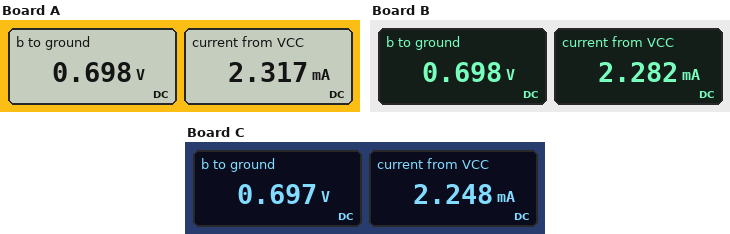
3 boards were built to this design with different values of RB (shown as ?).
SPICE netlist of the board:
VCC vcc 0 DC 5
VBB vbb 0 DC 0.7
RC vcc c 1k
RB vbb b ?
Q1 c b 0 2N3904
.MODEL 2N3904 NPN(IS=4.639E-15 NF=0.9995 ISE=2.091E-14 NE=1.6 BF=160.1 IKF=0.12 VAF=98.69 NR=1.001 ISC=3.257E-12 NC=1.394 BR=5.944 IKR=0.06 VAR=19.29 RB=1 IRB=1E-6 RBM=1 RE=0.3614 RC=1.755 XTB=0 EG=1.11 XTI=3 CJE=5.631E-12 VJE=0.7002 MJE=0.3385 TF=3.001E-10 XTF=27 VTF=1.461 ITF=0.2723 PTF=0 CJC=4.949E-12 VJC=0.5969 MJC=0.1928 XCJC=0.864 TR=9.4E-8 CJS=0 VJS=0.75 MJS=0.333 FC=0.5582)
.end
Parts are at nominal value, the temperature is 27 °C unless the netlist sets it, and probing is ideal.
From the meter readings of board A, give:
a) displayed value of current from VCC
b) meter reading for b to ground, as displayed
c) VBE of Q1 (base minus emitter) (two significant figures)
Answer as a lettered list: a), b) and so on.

a) 2.317 mA
b) 0.698 V
c) 700 mV
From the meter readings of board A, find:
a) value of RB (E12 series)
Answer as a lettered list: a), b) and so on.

a) 120 Ω
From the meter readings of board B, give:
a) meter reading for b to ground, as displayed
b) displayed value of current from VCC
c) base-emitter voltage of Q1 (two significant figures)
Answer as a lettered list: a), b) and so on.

a) 0.698 V
b) 2.282 mA
c) 700 mV
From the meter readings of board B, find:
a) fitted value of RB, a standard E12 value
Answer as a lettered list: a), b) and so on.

a) 150 Ω
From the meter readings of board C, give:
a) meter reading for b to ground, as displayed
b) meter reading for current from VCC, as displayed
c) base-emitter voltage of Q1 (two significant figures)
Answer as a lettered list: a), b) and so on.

a) 0.697 V
b) 2.248 mA
c) 700 mV
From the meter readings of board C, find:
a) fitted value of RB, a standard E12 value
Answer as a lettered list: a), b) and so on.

a) 180 Ω
